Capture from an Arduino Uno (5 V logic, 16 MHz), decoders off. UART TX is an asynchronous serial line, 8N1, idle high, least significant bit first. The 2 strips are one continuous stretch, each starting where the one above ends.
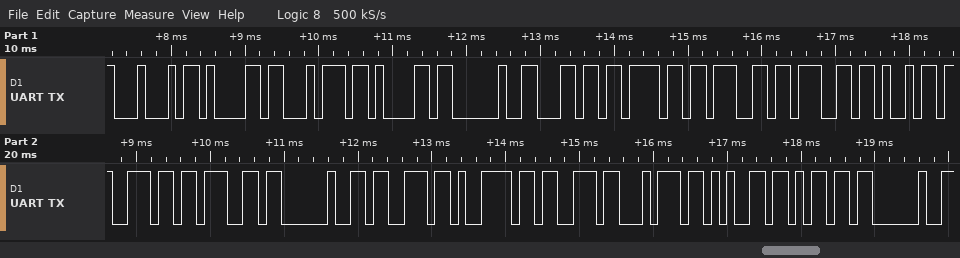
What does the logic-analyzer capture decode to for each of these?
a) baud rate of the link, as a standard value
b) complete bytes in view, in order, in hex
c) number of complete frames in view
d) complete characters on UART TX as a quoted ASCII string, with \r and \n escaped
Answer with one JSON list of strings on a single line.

["9600 baud", "44 61 74 61 20 6C 6F 67 67 69 6E 67 20 73 79 73 74 65 6D 20", "20", "\"Data logging system \""]
